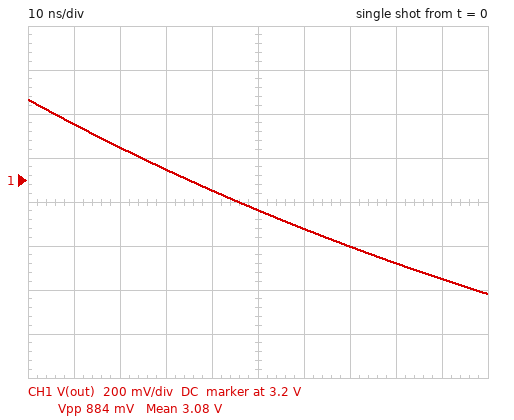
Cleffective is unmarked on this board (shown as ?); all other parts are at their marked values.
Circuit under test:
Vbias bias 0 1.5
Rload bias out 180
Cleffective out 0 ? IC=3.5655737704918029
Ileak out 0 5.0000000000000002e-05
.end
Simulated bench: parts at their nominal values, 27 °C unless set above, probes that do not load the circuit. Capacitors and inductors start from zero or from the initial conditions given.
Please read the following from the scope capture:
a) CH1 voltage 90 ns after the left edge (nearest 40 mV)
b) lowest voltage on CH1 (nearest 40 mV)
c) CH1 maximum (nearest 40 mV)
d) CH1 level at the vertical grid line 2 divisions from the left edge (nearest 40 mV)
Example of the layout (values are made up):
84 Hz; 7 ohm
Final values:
2.76 V; 2.68 V; 3.56 V; 3.36 V
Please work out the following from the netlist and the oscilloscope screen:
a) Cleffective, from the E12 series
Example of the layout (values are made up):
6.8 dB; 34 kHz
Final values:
1 nF
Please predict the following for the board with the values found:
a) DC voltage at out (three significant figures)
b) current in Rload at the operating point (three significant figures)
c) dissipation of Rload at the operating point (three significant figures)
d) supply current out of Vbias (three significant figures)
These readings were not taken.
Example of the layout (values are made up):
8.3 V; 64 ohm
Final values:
1.49 V; 50.0 µA; 450 nW; 50.0 µA
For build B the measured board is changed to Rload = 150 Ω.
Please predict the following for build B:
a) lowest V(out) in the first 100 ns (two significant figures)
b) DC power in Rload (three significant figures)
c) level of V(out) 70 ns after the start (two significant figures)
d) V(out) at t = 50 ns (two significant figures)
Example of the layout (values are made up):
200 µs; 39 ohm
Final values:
2.6 V; 375 nW; 2.8 V; 3.0 V
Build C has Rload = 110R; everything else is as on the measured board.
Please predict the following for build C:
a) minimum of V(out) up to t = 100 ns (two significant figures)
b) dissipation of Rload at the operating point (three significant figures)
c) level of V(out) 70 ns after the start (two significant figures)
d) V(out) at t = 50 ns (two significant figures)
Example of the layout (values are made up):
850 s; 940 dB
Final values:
2.3 V; 275 nW; 2.6 V; 2.8 V
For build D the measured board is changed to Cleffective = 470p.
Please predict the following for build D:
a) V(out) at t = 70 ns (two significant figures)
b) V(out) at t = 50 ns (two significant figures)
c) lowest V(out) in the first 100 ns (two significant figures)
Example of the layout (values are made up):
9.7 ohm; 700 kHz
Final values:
2.4 V; 2.6 V; 2.1 V
